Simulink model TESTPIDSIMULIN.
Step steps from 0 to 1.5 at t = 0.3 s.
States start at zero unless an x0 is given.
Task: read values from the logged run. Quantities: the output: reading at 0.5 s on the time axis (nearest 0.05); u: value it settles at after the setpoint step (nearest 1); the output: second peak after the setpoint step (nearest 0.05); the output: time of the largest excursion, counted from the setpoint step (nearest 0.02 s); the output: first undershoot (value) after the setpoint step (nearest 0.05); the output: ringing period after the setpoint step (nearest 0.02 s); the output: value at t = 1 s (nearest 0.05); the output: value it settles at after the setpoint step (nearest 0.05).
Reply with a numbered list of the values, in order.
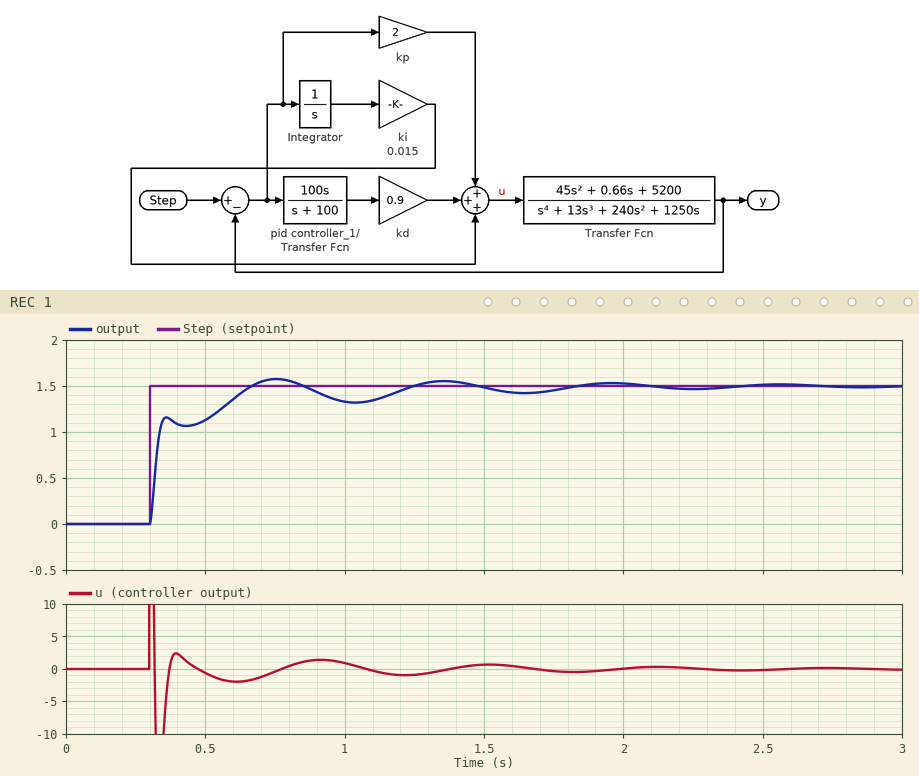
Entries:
1. 1.15
2. 0
3. 1.55
4. 0.46 s
5. 1.30
6. 0.60 s
7. 1.35
8. 1.50
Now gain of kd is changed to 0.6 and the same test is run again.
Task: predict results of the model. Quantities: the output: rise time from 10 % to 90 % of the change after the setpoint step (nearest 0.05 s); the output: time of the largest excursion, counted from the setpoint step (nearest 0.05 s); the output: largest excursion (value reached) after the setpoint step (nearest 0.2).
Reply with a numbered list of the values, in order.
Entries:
1. 0.30 s
2. 0.45 s
3. 1.6
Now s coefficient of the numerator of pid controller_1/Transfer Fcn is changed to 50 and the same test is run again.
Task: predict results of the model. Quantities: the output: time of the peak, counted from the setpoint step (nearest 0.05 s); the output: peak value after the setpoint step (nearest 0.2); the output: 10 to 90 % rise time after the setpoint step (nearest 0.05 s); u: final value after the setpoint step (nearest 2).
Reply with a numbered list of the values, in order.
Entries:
1. 0.50 s
2. 1.6
3. 0.30 s
4. 0
